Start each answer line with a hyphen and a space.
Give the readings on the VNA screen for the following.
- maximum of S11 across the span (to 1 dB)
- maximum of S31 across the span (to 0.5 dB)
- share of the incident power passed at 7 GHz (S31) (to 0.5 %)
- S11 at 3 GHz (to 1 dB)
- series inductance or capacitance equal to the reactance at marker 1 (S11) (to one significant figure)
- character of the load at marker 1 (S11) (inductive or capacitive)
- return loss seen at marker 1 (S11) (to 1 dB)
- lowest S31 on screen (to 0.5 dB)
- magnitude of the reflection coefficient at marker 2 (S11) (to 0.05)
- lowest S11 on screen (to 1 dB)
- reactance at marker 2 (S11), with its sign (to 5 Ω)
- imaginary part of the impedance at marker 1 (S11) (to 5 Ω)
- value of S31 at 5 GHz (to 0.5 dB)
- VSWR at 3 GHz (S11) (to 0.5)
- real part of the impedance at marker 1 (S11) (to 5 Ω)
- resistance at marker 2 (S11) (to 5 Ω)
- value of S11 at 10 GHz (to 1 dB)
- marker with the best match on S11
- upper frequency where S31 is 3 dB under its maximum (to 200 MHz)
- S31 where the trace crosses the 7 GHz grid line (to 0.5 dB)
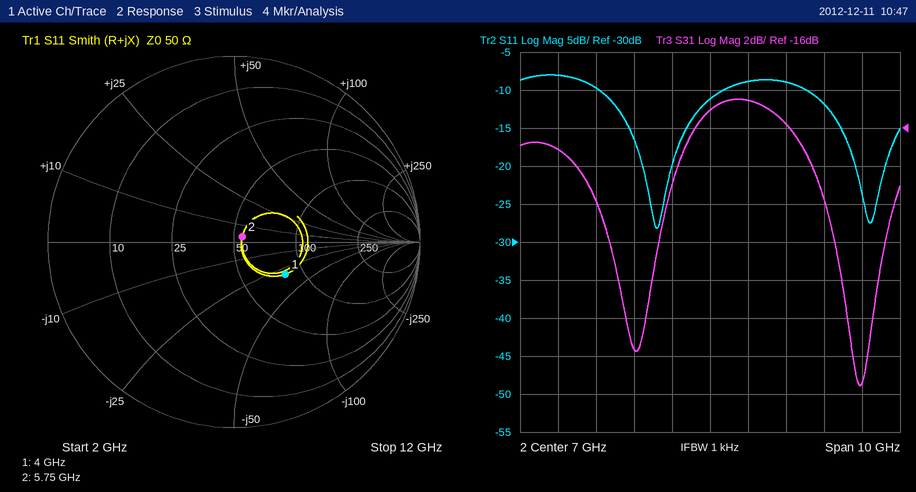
- -8 dB
- -14.5 dB
- 3.0 %
- -8 dB
- 1 pF
- capacitive
- 10 dB
- -29.5 dB
- 0.05
- -28 dB
- +5 Ω
- -30 Ω
- -27.5 dB
- 2.5
- 80 Ω
- 55 Ω
- -12 dB
- marker 2
- 9.6 GHz
- -15.0 dB
